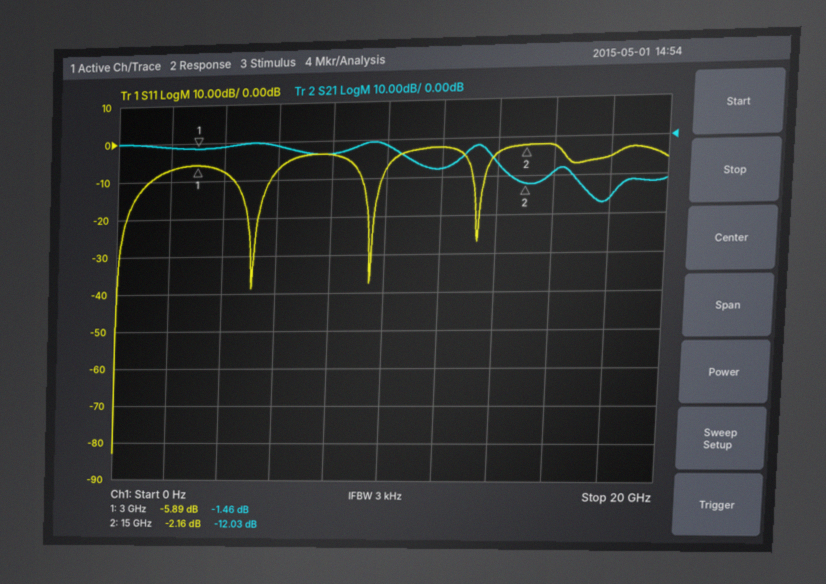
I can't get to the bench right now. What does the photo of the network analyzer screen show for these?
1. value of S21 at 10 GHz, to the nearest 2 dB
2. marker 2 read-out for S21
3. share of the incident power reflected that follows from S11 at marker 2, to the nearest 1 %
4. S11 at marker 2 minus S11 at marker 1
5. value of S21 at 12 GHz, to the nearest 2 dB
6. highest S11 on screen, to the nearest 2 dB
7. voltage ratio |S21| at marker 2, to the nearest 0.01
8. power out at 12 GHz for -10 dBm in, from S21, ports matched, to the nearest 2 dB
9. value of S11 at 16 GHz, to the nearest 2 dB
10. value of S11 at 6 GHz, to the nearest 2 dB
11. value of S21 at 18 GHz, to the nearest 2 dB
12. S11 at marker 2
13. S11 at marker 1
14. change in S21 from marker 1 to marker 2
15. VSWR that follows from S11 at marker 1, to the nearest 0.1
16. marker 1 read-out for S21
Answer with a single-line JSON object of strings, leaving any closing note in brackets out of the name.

{"value of S21 at 10 GHz, to the nearest 2 dB": "-2 dB", "marker 2 read-out for S21": "-12.03 dB", "share of the incident power reflected that follows from S11 at marker 2, to the nearest 1 %": "61 %", "S11 at marker 2 minus S11 at marker 1": "3.73 dB", "value of S21 at 12 GHz, to the nearest 2 dB": "-8 dB", "highest S11 on screen, to the nearest 2 dB": "-2 dB", "voltage ratio |S21| at marker 2, to the nearest 0.01": "0.25", "power out at 12 GHz for -10 dBm in, from S21, ports matched, to the nearest 2 dB": "-18 dBm", "value of S11 at 16 GHz, to the nearest 2 dB": "-2 dB", "value of S11 at 6 GHz, to the nearest 2 dB": "-8 dB", "value of S21 at 18 GHz, to the nearest 2 dB": "-16 dB", "S11 at marker 2": "-2.16 dB", "S11 at marker 1": "-5.89 dB", "change in S21 from marker 1 to marker 2": "-10.57 dB", "VSWR that follows from S11 at marker 1, to the nearest 0.1": "3.1", "marker 1 read-out for S21": "-1.46 dB"}
